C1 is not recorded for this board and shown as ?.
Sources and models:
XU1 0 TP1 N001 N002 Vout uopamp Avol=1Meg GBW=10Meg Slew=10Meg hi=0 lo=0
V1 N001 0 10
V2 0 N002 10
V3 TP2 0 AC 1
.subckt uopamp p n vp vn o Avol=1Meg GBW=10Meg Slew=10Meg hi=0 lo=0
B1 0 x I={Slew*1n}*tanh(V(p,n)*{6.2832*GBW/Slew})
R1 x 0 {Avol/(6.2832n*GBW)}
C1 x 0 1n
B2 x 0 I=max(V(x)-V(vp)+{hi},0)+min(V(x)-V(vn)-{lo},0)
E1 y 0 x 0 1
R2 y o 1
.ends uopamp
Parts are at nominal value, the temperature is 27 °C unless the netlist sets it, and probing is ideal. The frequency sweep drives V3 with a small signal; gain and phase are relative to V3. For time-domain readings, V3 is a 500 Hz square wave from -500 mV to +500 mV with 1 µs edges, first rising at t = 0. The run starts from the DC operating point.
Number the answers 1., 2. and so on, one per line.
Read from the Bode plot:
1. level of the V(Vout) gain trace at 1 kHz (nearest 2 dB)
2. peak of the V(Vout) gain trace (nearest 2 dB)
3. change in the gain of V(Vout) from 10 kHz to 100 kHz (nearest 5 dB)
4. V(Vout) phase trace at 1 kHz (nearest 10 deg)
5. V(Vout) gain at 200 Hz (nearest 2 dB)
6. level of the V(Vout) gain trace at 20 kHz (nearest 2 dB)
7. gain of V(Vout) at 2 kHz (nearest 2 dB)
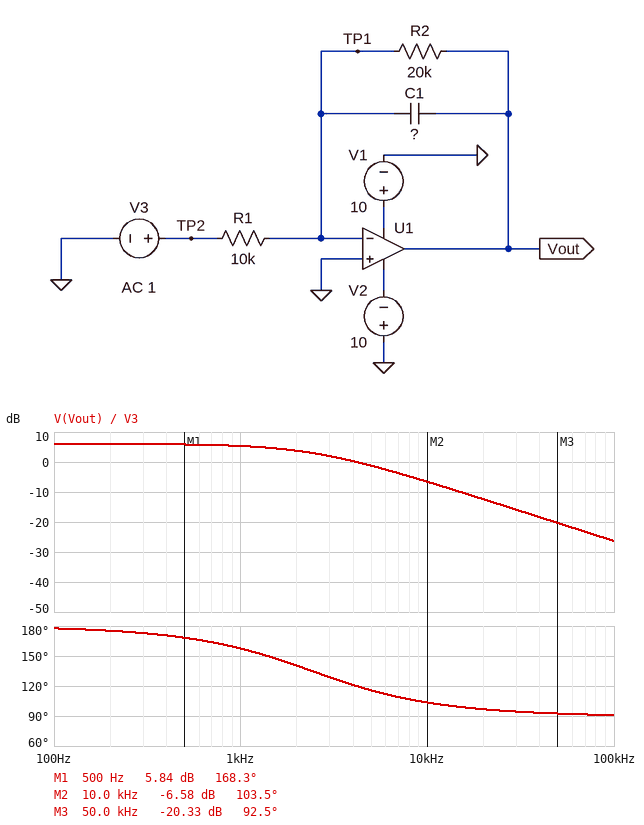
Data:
1. 6 dB
2. 6 dB
3. -20 dB
4. 160 deg
5. 6 dB
6. -12 dB
7. 4 dB
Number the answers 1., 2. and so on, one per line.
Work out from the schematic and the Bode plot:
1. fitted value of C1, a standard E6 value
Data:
1. 3.3 nF
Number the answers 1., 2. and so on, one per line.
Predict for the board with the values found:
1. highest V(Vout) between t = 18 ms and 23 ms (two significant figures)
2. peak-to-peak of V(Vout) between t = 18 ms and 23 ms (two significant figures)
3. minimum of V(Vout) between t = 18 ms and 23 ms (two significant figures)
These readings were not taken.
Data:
1. 1.0 V
2. 2.0 V
3. -1.0 V
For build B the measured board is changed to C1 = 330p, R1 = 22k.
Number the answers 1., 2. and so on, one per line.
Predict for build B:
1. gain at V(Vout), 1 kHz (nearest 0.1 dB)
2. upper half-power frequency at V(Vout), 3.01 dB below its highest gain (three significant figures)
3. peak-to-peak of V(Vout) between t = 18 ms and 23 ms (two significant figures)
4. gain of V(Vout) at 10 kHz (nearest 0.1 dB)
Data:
1. -0.8 dB
2. 24.1 kHz
3. 910 mV
4. -1.5 dB
